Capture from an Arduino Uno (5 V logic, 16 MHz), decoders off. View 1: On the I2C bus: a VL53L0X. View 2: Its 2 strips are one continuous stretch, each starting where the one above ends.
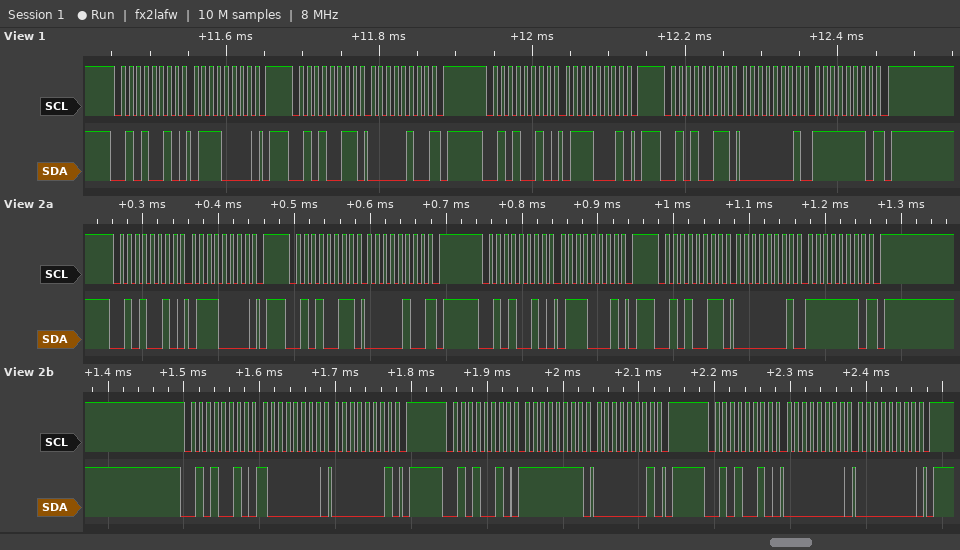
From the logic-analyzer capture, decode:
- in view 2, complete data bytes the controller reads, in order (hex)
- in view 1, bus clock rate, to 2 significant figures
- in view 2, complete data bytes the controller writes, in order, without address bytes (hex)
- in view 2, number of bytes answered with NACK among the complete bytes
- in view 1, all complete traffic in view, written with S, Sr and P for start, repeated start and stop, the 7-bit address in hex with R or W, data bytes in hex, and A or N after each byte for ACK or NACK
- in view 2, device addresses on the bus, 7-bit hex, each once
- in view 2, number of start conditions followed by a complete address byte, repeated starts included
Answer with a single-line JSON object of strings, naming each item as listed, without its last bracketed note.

{"in view 2, complete data bytes the controller reads, in order": "04 01 FE", "in view 1, bus clock rate, to 2 significant figures": "100 kHz", "in view 2, complete data bytes the controller writes, in order, without address bytes": "70 71 80 01 FF 01 00 00", "in view 2, number of bytes answered with NACK among the complete bytes": "2", "in view 1, all complete traffic in view, written with S, Sr and P for start, repeated start and stop, the 7-bit address in hex with R or W, data bytes in hex, and A or N after each byte for ACK or NACK": "S 29W A 70 A P S 29R A 04 N P S 29W A 71 A P S 29R A 01 A FE N P", "in view 2, device addresses on the bus, 7-bit hex, each once": "0x29", "in view 2, number of start conditions followed by a complete address byte, repeated starts included": "7"}
